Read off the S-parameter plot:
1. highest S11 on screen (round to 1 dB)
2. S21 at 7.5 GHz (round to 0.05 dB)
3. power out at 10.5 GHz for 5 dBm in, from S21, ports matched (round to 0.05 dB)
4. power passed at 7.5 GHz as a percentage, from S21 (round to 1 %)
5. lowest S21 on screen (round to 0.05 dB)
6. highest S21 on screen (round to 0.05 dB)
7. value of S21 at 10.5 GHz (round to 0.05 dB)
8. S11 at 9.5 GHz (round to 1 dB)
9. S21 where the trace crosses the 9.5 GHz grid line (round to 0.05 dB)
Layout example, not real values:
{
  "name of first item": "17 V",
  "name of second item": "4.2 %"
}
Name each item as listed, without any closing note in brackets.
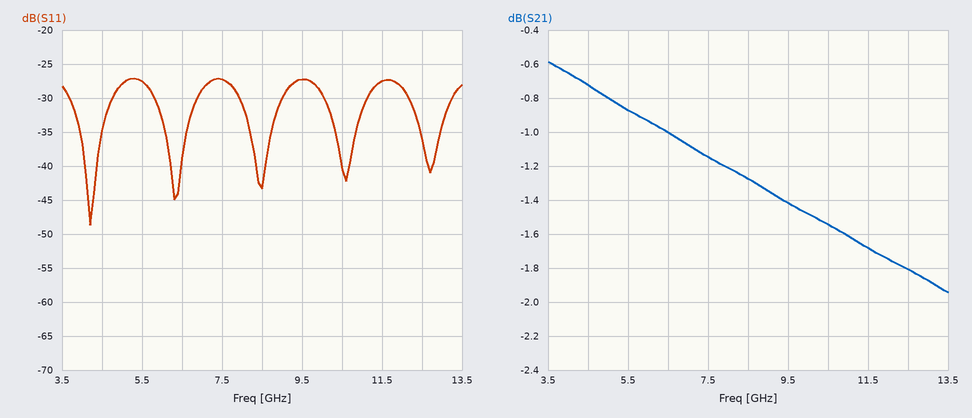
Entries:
{
  "highest S11 on screen": "-27 dB",
  "S21 at 7.5 GHz": "-1.15 dB",
  "power out at 10.5 GHz for 5 dBm in, from S21, ports matched": "3.45 dBm",
  "power passed at 7.5 GHz as a percentage, from S21": "77 %",
  "lowest S21 on screen": "-1.95 dB",
  "highest S21 on screen": "-0.60 dB",
  "value of S21 at 10.5 GHz": "-1.55 dB",
  "S11 at 9.5 GHz": "-27 dB",
  "S21 where the trace crosses the 9.5 GHz grid line": "-1.40 dB"
}
